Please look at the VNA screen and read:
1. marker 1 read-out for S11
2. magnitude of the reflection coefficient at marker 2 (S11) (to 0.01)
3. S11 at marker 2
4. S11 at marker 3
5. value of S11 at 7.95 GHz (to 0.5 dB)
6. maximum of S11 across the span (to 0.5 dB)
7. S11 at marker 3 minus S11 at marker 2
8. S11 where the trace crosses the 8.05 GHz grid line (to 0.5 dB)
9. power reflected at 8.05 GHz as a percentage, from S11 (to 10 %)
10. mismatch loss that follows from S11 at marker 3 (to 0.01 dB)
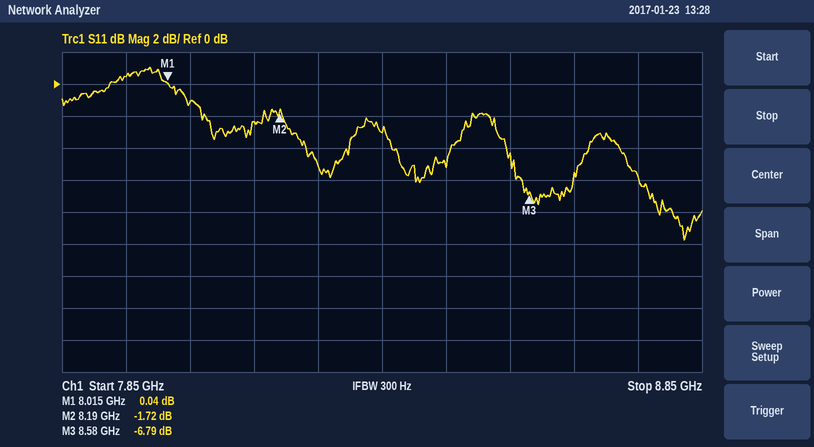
0.04 dB
0.82
-1.72 dB
-6.79 dB
0.5 dB
1.0 dB
-5.07 dB
-1.0 dB
80 %
1.02 dB
